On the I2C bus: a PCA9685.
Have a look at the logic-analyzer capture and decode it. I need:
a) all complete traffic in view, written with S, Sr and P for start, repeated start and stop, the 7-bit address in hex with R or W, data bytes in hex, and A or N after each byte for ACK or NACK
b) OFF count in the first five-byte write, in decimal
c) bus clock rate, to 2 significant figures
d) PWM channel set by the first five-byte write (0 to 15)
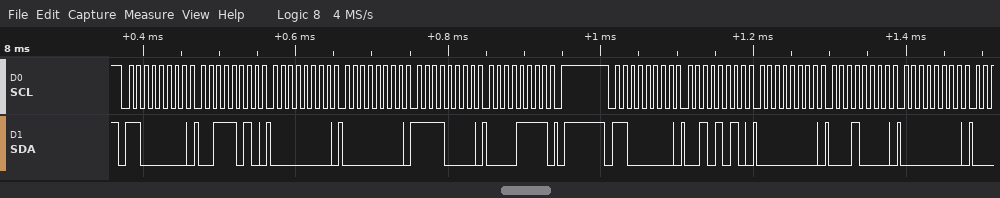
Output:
S 60W A 3A A 00 A 00 A F0 A 0F A P S 60W A 2A A 00 A 10 A 00 A
4080
100 kHz
13
